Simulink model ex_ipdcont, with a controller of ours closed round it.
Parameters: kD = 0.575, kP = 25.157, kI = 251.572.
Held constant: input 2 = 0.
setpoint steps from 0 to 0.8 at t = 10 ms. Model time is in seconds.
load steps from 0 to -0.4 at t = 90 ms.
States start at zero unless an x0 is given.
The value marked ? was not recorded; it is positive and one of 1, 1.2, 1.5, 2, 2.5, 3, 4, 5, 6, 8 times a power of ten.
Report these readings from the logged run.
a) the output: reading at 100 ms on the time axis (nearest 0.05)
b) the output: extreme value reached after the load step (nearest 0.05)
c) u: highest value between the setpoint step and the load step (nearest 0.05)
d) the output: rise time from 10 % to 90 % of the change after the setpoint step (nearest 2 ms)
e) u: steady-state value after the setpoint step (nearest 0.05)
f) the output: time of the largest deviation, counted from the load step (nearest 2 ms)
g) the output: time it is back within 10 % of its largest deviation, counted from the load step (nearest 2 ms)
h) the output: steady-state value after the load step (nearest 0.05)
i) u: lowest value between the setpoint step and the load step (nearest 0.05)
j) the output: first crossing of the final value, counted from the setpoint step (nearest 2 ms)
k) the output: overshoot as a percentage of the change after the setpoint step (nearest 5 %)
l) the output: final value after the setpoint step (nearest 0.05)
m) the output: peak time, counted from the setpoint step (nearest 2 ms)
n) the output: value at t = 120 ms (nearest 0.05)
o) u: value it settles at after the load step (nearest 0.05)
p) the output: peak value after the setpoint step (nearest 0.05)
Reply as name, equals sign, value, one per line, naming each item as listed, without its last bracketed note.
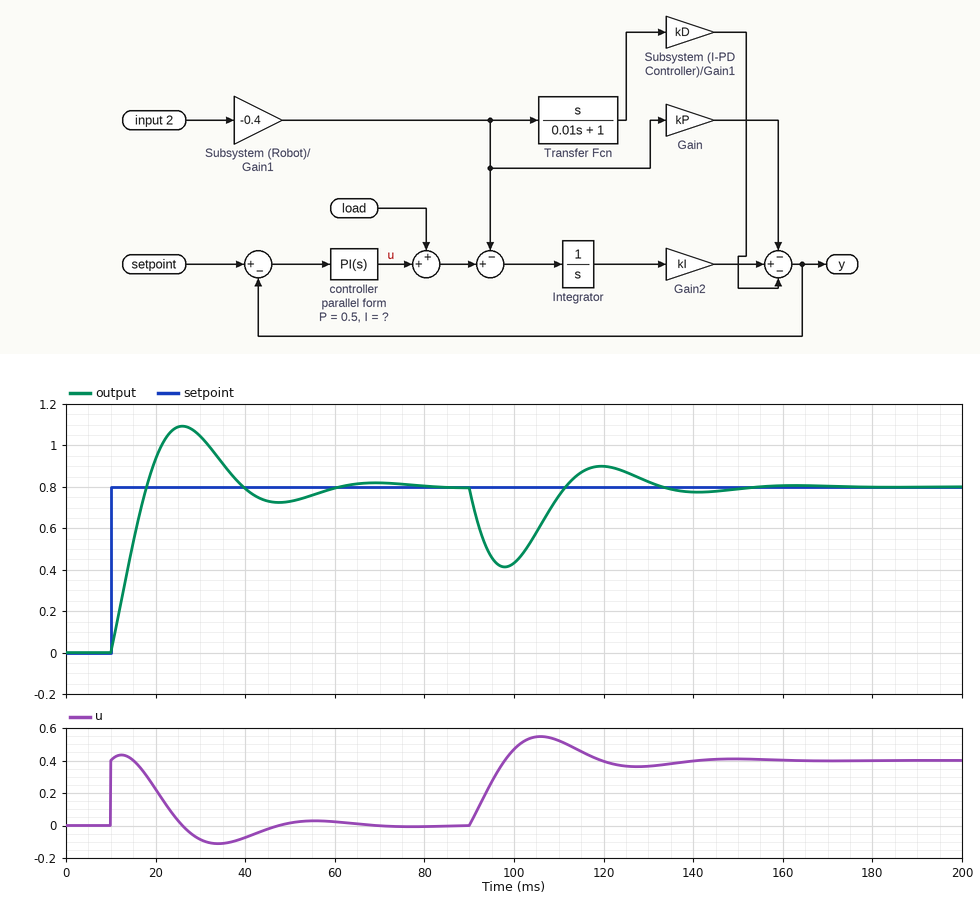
the output: reading at 100 ms on the time axis = 0.45
the output: extreme value reached after the load step = 0.40
u: highest value between the setpoint step and the load step = 0.45
the output: rise time from 10 % to 90 % of the change after the setpoint step = 6 ms
u: steady-state value after the setpoint step = 0.00
the output: time of the largest deviation, counted from the load step = 8 ms
the output: time it is back within 10 % of its largest deviation, counted from the load step = 38 ms
the output: steady-state value after the load step = 0.80
u: lowest value between the setpoint step and the load step = -0.10
the output: first crossing of the final value, counted from the setpoint step = 8 ms
the output: overshoot as a percentage of the change after the setpoint step = 35 %
the output: final value after the setpoint step = 0.80
the output: peak time, counted from the setpoint step = 16 ms
the output: value at t = 120 ms = 0.90
u: value it settles at after the load step = 0.40
the output: peak value after the setpoint step = 1.10
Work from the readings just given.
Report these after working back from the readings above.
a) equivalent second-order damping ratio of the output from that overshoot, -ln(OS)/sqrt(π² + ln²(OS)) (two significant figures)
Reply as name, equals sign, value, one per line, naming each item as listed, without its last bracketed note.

equivalent second-order damping ratio of the output from that overshoot, -ln(OS)/sqrt(π² + ln²(OS)) = 0.32
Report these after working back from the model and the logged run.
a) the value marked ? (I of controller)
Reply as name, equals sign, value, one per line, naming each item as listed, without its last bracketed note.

the value marked ? = 100
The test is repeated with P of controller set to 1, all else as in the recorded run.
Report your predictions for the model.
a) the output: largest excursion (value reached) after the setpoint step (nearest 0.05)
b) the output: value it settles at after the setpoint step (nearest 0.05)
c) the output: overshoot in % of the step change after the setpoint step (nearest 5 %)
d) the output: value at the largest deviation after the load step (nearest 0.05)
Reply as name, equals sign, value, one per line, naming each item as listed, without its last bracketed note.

the output: largest excursion (value reached) after the setpoint step = 0.95
the output: value it settles at after the setpoint step = 0.80
the output: overshoot in % of the step change after the setpoint step = 20 %
the output: value at the largest deviation after the load step = 0.55
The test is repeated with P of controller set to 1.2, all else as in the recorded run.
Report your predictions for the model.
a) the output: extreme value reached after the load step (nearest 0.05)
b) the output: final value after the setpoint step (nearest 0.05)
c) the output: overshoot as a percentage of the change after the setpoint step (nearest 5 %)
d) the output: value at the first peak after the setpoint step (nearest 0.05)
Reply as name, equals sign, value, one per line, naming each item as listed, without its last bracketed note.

the output: extreme value reached after the load step = 0.55
the output: final value after the setpoint step = 0.80
the output: overshoot as a percentage of the change after the setpoint step = 15 %
the output: value at the first peak after the setpoint step = 0.90
